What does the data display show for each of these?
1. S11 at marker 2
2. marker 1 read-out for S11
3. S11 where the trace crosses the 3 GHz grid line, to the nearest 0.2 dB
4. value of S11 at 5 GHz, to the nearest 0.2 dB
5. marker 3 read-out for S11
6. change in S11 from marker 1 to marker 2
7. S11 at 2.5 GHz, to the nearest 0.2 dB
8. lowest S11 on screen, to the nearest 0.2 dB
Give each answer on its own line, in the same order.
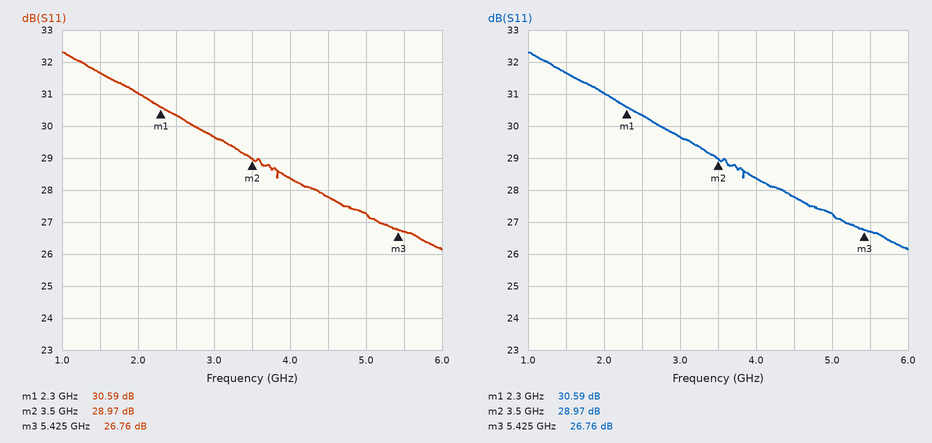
28.97 dB
30.59 dB
29.6 dB
27.2 dB
26.76 dB
-1.62 dB
30.4 dB
26.2 dB
